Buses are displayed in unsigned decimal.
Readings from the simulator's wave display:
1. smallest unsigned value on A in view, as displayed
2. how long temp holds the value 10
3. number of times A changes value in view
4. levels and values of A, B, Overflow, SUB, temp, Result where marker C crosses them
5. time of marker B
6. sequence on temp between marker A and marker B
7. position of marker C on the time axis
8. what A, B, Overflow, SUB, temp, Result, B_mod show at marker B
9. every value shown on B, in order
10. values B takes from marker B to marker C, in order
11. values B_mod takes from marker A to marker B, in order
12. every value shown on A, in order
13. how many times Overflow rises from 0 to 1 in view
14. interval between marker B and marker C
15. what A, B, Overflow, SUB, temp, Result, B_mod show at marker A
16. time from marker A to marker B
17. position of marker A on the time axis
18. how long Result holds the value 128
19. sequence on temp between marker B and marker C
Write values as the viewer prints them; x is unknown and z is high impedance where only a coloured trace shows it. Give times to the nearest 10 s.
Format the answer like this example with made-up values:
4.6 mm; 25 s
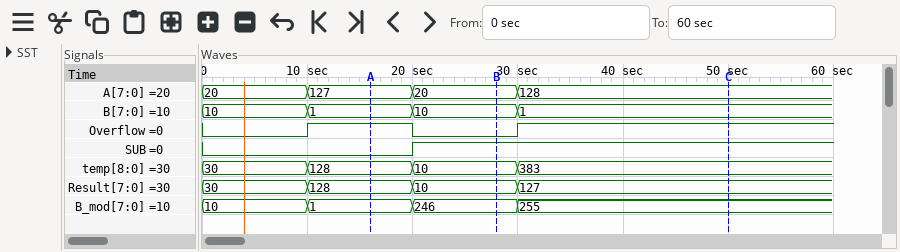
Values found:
20; 10 s; 3; A=128, B=1, Overflow=1, SUB=1, temp=383, Result=127; 30 s; 128, 10; 50 s; A=20, B=10, Overflow=0, SUB=1, temp=10, Result=10, B_mod=246; 10, 1, 10, 1; 10, 1; 1, 246; 20, 127, 20, 128; 2; 20 s; A=127, B=1, Overflow=1, SUB=0, temp=128, Result=128, B_mod=1; 10 s; 20 s; 10 s; 10, 383
